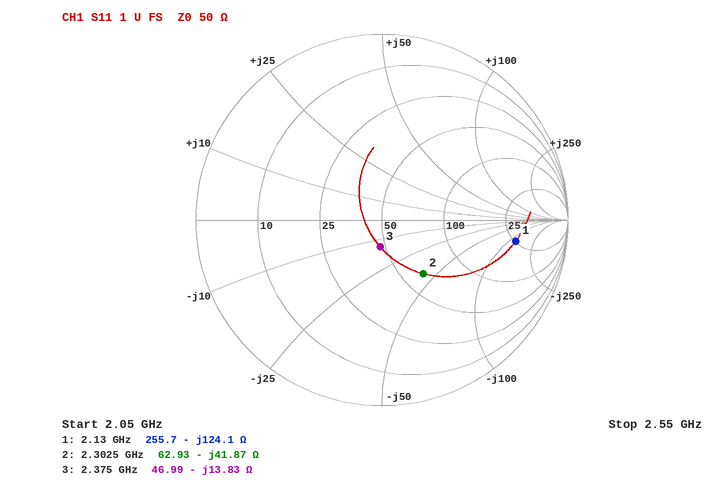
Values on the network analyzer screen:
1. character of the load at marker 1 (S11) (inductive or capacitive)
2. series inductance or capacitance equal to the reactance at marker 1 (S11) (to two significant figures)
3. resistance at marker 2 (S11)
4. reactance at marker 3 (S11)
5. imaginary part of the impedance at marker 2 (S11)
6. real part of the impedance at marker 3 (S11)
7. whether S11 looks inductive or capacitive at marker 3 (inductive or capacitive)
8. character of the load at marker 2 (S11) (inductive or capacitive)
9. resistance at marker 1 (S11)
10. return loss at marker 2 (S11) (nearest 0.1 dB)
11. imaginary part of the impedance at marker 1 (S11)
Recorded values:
capacitive
600 fF
62.93 Ω
-13.83 Ω
-41.87 Ω
46.99 Ω
capacitive
capacitive
255.7 Ω
8.8 dB
-124.1 Ω
